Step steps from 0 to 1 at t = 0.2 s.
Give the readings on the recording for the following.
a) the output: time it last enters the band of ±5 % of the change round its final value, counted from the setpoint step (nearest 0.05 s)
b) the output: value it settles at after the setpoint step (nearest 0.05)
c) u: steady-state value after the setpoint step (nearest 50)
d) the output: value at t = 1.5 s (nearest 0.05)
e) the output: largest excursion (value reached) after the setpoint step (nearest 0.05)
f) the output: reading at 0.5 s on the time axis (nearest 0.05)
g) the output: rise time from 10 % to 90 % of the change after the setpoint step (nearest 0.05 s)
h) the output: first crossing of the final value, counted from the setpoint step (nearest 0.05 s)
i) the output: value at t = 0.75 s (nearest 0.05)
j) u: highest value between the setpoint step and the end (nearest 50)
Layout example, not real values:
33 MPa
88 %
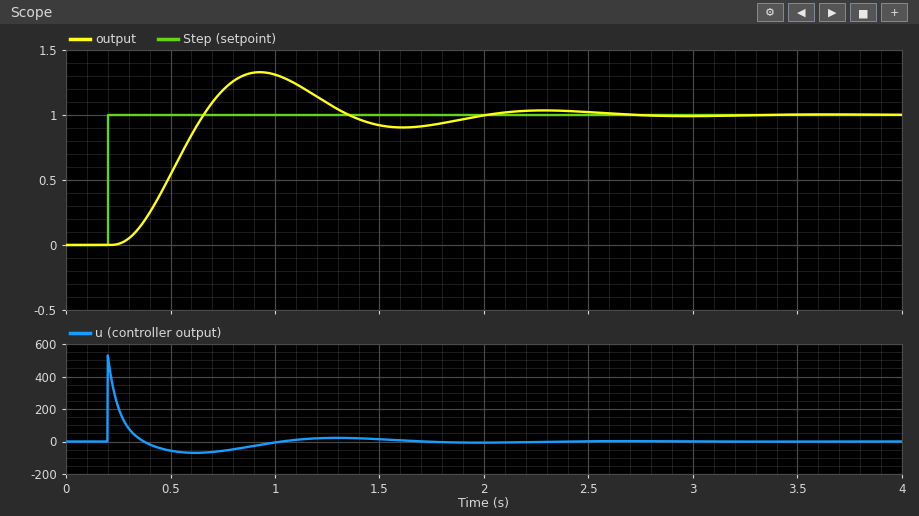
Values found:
1.65 s
1.00
0
0.90
1.35
0.55
0.30 s
0.45 s
1.20
550
